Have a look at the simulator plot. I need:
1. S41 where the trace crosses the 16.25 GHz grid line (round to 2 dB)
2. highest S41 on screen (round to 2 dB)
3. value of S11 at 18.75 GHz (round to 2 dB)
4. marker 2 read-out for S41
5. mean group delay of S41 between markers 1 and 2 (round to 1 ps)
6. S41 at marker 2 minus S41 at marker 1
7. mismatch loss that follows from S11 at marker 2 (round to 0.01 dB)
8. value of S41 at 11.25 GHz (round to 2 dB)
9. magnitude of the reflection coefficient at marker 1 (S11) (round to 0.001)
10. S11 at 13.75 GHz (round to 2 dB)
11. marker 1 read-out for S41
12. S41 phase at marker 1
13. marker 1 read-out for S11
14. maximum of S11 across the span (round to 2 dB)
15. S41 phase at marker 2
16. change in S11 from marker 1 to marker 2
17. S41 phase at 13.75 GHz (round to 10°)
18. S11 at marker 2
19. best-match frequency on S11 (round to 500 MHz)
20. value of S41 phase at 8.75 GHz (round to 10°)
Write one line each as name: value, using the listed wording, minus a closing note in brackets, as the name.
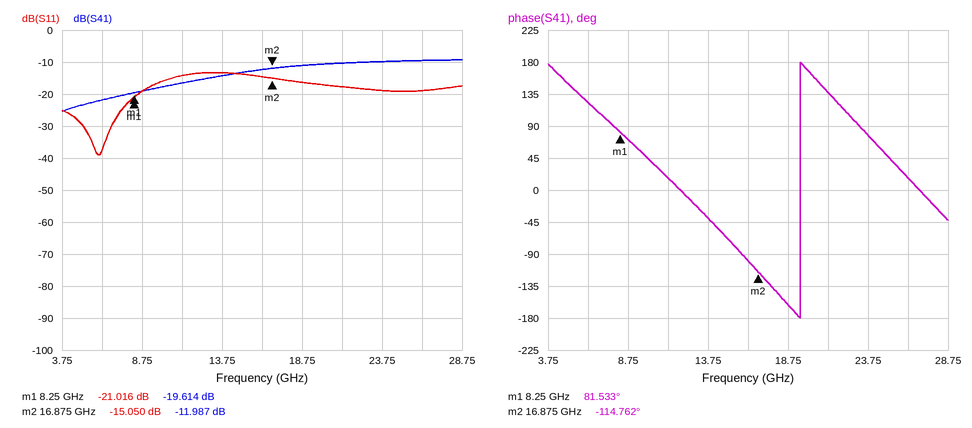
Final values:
S41 where the trace crosses the 16.25 GHz grid line: -12 dB
highest S41 on screen: -10 dB
value of S11 at 18.75 GHz: -16 dB
marker 2 read-out for S41: -11.987 dB
mean group delay of S41 between markers 1 and 2: 63 ps
S41 at marker 2 minus S41 at marker 1: 7.627 dB
mismatch loss that follows from S11 at marker 2: 0.14 dB
value of S41 at 11.25 GHz: -16 dB
magnitude of the reflection coefficient at marker 1 (S11): 0.089
S11 at 13.75 GHz: -14 dB
marker 1 read-out for S41: -19.614 dB
S41 phase at marker 1: 81.533°
marker 1 read-out for S11: -21.016 dB
maximum of S11 across the span: -14 dB
S41 phase at marker 2: -114.762°
change in S11 from marker 1 to marker 2: 5.966 dB
S41 phase at 13.75 GHz: -40°
S11 at marker 2: -15.050 dB
best-match frequency on S11: 6.0 GHz
value of S41 phase at 8.75 GHz: 70°
